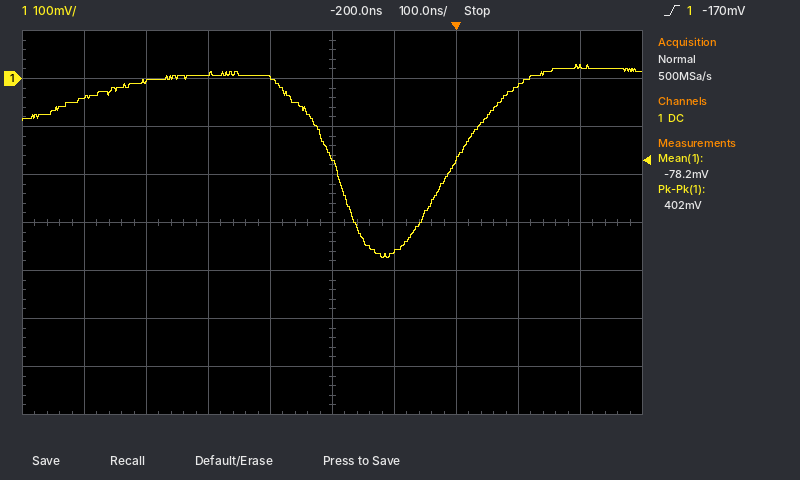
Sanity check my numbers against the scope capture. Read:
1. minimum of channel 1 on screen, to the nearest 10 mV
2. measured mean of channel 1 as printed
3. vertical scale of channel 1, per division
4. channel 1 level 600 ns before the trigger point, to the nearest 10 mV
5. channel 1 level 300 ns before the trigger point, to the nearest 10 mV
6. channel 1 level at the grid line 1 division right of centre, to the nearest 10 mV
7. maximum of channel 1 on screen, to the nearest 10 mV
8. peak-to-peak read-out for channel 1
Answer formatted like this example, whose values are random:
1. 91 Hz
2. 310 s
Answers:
1. -370 mV
2. -78.2 mV
3. 100 mV
4. -40 mV
5. 0 mV
6. -360 mV
7. 30 mV
8. 402 mV
